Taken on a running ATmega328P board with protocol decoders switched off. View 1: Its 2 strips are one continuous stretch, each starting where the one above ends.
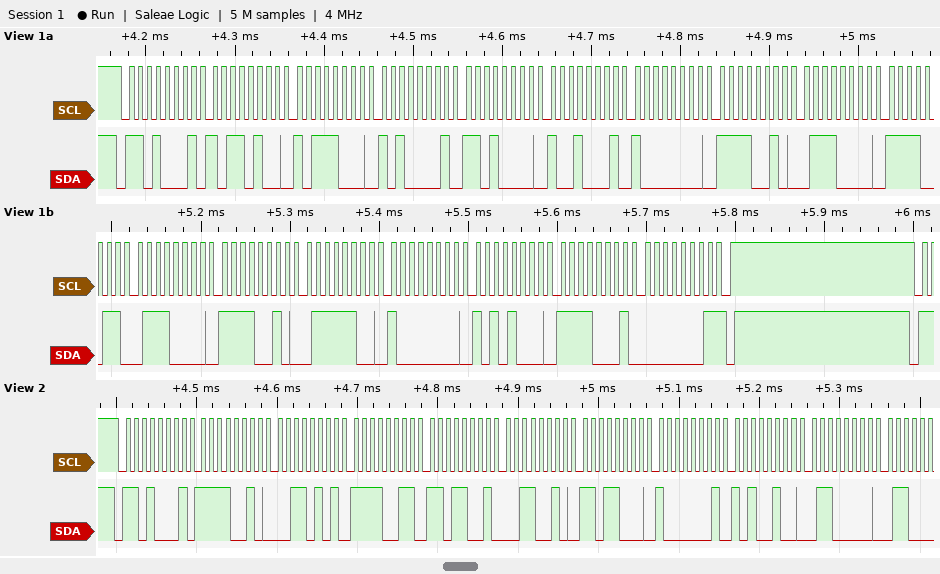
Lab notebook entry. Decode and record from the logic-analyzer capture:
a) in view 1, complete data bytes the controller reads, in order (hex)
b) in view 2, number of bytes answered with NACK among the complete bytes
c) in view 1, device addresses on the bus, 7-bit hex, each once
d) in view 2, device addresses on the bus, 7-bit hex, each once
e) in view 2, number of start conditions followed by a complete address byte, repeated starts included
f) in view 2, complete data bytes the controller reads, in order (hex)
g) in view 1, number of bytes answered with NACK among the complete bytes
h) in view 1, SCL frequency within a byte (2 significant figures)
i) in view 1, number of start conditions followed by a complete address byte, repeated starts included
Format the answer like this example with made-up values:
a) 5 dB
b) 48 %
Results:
a) B4 B8 A1 D0 91 80 F2 70 F3 70 F2 7C 80 A8 F1 01
b) 0
c) 0x68
d) 0x68
e) 1
f) F2 35 F3 D9 32 D8 81 A4 60
g) 1
h) 100 kHz
i) 1
